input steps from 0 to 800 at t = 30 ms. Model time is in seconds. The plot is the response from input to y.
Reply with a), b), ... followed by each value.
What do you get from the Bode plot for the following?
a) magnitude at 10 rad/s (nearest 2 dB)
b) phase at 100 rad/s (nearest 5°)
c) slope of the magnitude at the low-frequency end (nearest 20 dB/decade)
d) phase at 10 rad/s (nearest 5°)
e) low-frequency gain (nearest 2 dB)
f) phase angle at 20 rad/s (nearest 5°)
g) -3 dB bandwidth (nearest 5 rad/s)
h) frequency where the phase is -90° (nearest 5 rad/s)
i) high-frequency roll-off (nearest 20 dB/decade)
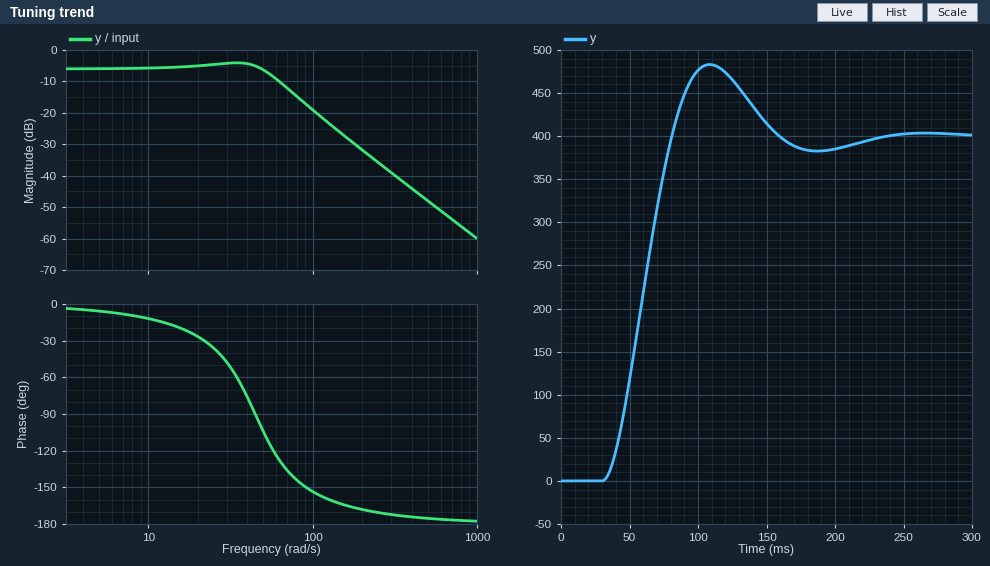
a) -6 dB
b) -155°
c) 0 dB/decade
d) -10°
e) -6 dB
f) -25°
g) 60 rad/s
h) 45 rad/s
i) -40 dB/decade
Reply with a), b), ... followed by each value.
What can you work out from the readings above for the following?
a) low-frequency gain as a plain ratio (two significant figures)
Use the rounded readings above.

a) 0.50
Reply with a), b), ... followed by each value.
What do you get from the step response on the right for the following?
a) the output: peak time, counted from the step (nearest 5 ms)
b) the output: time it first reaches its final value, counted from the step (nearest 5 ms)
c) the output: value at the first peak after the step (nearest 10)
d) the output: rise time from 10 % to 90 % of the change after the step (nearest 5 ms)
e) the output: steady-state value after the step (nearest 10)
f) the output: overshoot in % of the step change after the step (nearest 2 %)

a) 80 ms
b) 50 ms
c) 480
d) 35 ms
e) 400
f) 20 %
